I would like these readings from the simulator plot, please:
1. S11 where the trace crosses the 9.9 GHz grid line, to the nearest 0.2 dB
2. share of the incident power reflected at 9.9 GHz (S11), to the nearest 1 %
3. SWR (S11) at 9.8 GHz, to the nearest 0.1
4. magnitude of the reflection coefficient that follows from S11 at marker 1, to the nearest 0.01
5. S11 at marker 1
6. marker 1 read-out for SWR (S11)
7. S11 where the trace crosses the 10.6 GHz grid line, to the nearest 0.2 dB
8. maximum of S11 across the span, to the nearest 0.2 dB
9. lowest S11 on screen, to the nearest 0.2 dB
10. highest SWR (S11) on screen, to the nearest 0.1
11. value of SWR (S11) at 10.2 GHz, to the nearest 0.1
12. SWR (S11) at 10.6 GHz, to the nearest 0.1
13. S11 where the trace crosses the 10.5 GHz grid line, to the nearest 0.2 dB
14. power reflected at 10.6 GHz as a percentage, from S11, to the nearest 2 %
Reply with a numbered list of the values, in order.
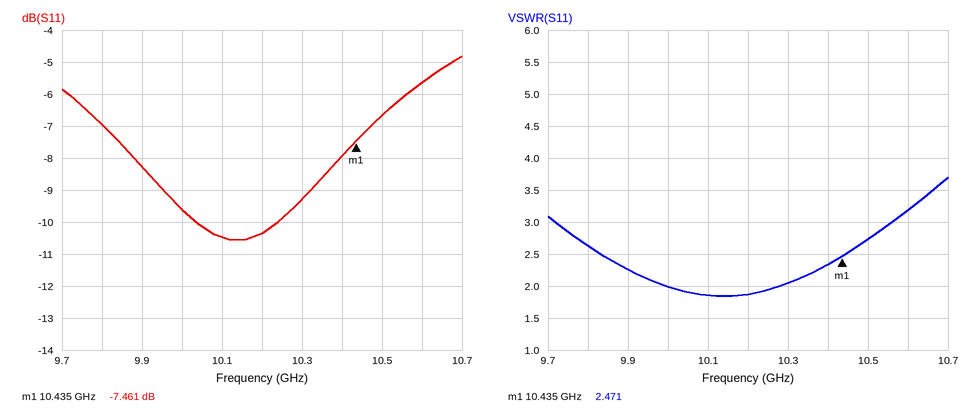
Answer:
1. -8.2 dB
2. 15 %
3. 2.6
4. 0.42
5. -7.461 dB
6. 2.471
7. -5.6 dB
8. -4.8 dB
9. -10.6 dB
10. 3.7
11. 1.9
12. 3.2
13. -6.6 dB
14. 28 %
